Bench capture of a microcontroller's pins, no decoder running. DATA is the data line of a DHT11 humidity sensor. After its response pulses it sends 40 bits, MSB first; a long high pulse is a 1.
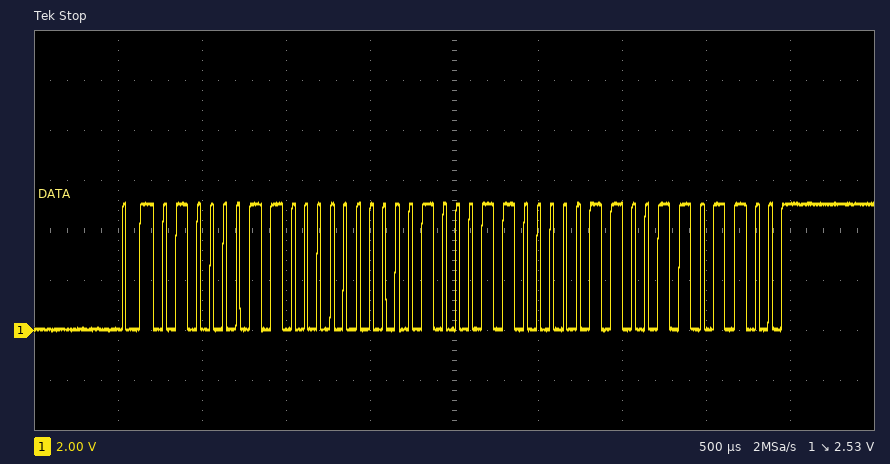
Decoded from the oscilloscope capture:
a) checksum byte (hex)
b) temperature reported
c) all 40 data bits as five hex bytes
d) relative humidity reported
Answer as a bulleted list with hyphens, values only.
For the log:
- 0x6C
- 35.6 °C
- 43 00 23 06 6C
- 67 %
